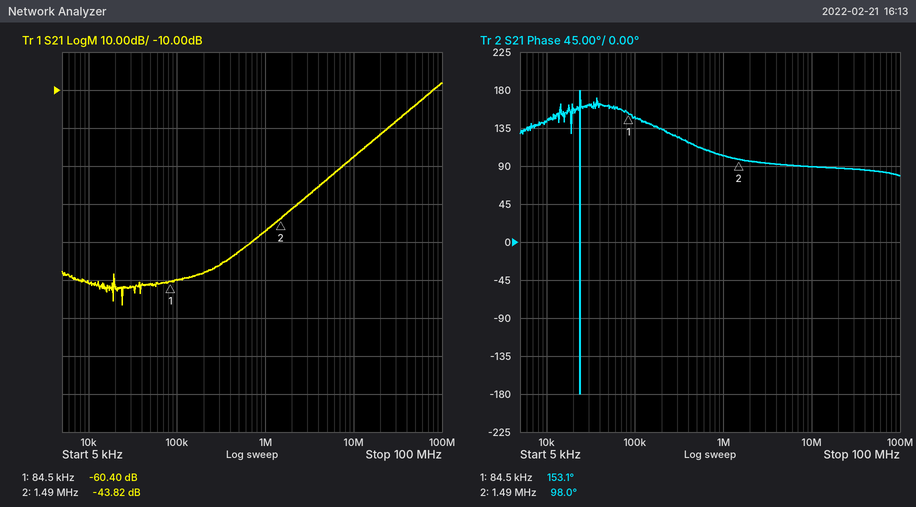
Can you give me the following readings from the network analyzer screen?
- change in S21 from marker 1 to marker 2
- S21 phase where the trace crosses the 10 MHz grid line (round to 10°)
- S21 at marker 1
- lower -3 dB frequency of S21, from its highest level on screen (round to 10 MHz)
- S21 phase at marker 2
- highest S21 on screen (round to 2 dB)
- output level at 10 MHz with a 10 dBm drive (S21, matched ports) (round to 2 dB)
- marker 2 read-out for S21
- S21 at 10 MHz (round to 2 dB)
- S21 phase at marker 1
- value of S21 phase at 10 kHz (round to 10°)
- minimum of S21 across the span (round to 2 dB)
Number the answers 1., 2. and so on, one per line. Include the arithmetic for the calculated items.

1. -43.82 − (-60.4) = 16.58 dB
2. 90°
3. -60.40 dB
4. 70 MHz
5. 98.0°
6. -8 dB
7. 10 dBm + (-28 dB) = -18 dBm
8. -43.82 dB
9. -28 dB
10. 153.1°
11. 140°
12. -66 dB
